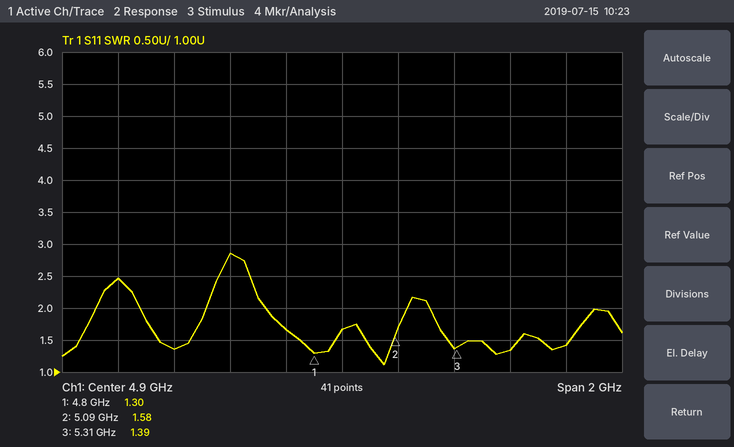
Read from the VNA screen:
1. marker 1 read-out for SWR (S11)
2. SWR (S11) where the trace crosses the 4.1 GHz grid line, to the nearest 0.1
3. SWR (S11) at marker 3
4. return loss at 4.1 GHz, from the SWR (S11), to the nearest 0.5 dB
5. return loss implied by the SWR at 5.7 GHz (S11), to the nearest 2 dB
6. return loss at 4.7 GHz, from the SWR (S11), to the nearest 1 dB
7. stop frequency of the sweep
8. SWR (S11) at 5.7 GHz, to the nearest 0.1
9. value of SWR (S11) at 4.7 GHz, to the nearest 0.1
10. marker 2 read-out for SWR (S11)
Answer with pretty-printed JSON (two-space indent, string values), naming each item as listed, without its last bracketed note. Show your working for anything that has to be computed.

{
  "marker 1 read-out for SWR": "1.30",
  "SWR (S11) where the trace crosses the 4.1 GHz grid line, to the nearest 0.1": "2.5",
  "SWR (S11) at marker 3": "1.39",
  "return loss at 4.1 GHz, from the SWR (S11), to the nearest 0.5 dB": "−20 log10((2.5 − 1)/(2.5 + 1)) ≈ 7.36 dB, so 7.5 dB to the nearest 0.5 dB",
  "return loss implied by the SWR at 5.7 GHz (S11), to the nearest 2 dB": "−20 log10((1.4 − 1)/(1.4 + 1)) ≈ 16 dB",
  "return loss at 4.7 GHz, from the SWR (S11), to the nearest 1 dB": "−20 log10((1.7 − 1)/(1.7 + 1)) ≈ 12 dB",
  "stop frequency of the sweep": "5.9 GHz",
  "SWR (S11) at 5.7 GHz, to the nearest 0.1": "1.4",
  "value of SWR (S11) at 4.7 GHz, to the nearest 0.1": "1.7",
  "marker 2 read-out for SWR": "1.58"
}
